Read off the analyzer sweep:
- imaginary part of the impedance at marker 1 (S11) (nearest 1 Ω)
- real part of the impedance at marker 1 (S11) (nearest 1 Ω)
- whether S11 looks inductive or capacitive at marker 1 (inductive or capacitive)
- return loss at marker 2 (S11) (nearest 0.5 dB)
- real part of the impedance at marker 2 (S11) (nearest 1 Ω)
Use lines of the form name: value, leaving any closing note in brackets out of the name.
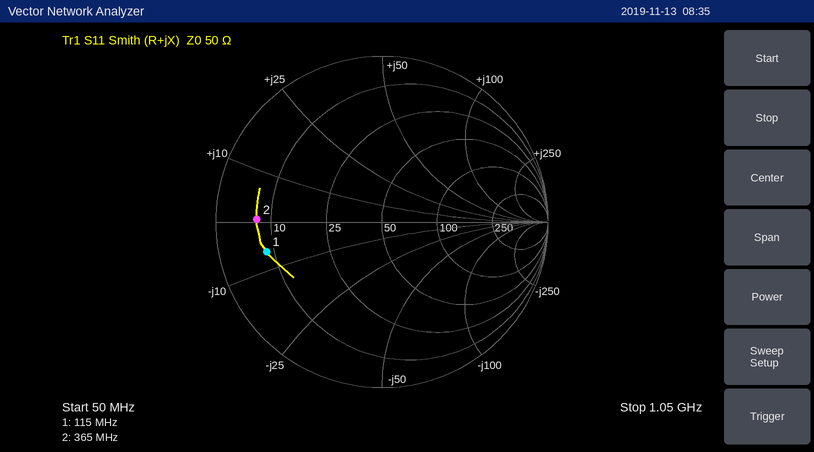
imaginary part of the impedance at marker 1 (S11): -6 Ω
real part of the impedance at marker 1 (S11): 8 Ω
whether S11 looks inductive or capacitive at marker 1: capacitive
return loss at marker 2 (S11): 2.5 dB
real part of the impedance at marker 2 (S11): 7 Ω
